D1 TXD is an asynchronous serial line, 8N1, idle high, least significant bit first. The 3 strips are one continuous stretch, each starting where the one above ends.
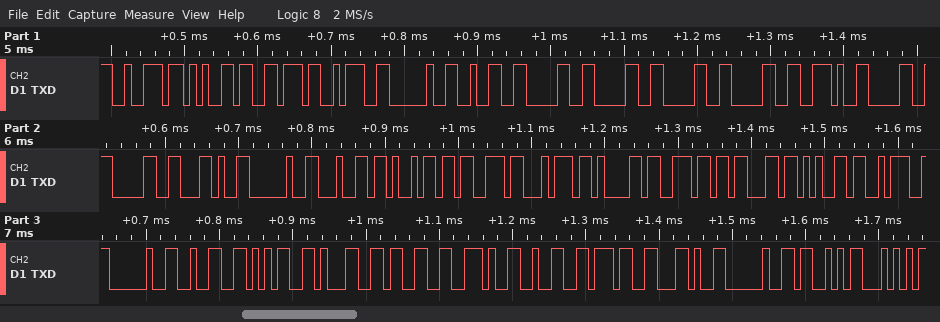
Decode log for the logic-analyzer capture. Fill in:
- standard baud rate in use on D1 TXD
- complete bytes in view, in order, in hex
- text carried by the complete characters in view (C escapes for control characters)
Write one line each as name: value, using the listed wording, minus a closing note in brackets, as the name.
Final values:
standard baud rate in use on D1 TXD: 115200 baud
complete bytes in view, in order, in hex: 72 65 76 3A 20 32 30 30 30 30 2E 30 30 2C 20 64 69 73 74 61 6E 63 65 3A 20 32 35 31 33 2E 32 37 2C 20 53 54
text carried by the complete characters in view: "rev: 20000.00, distance: 2513.27, ST"
